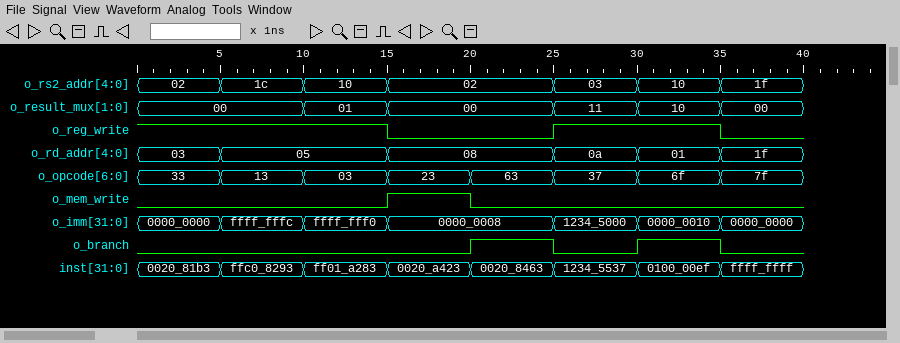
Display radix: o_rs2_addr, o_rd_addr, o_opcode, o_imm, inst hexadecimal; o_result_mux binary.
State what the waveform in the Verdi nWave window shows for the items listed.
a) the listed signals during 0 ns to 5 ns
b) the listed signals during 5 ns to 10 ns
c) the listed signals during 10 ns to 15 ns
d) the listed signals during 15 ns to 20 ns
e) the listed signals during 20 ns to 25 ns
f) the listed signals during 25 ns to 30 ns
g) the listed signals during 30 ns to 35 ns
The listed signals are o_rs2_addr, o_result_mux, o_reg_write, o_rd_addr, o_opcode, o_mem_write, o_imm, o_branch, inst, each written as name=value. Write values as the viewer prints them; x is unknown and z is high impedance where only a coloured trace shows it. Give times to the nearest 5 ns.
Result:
o_rs2_addr=02, o_result_mux=00, o_reg_write=1, o_rd_addr=03, o_opcode=33, o_mem_write=0, o_imm=0000_0000, o_branch=0, inst=0020_81b3
o_rs2_addr=1c, o_result_mux=00, o_reg_write=1, o_rd_addr=05, o_opcode=13, o_mem_write=0, o_imm=ffff_fffc, o_branch=0, inst=ffc0_8293
o_rs2_addr=10, o_result_mux=01, o_reg_write=1, o_rd_addr=05, o_opcode=03, o_mem_write=0, o_imm=ffff_fff0, o_branch=0, inst=ff01_a283
o_rs2_addr=02, o_result_mux=00, o_reg_write=0, o_rd_addr=08, o_opcode=23, o_mem_write=1, o_imm=0000_0008, o_branch=0, inst=0020_a423
o_rs2_addr=02, o_result_mux=00, o_reg_write=0, o_rd_addr=08, o_opcode=63, o_mem_write=0, o_imm=0000_0008, o_branch=1, inst=0020_8463
o_rs2_addr=03, o_result_mux=11, o_reg_write=1, o_rd_addr=0a, o_opcode=37, o_mem_write=0, o_imm=1234_5000, o_branch=0, inst=1234_5537
o_rs2_addr=10, o_result_mux=10, o_reg_write=1, o_rd_addr=01, o_opcode=6f, o_mem_write=0, o_imm=0000_0010, o_branch=1, inst=0100_00ef
